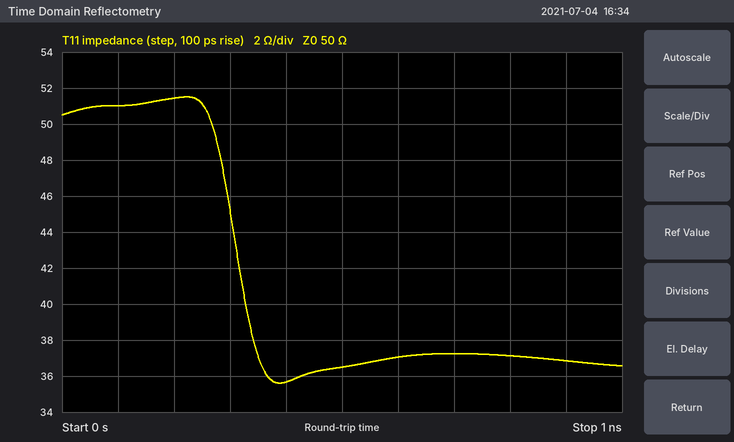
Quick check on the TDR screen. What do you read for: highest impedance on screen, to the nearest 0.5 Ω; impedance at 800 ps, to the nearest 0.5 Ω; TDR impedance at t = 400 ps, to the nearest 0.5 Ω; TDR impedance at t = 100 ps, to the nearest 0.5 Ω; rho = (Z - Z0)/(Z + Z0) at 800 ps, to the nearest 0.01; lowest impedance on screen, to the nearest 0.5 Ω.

51.5 Ω
37.0 Ω
35.5 Ω
51.0 Ω
-0.15
35.5 Ω
